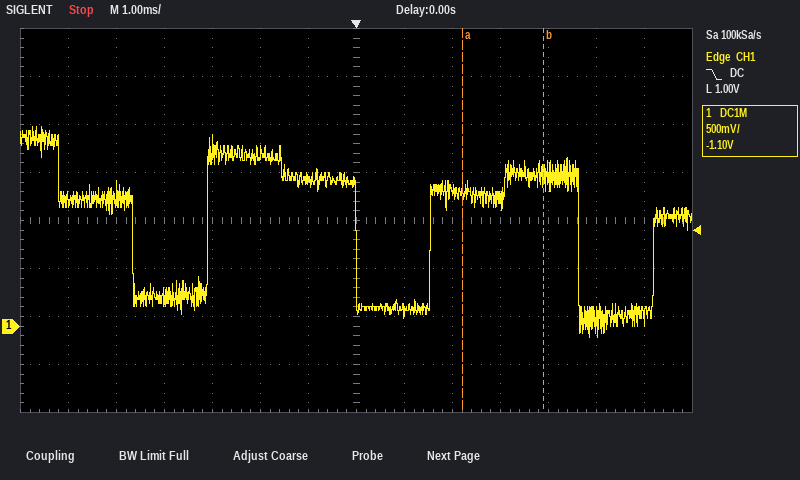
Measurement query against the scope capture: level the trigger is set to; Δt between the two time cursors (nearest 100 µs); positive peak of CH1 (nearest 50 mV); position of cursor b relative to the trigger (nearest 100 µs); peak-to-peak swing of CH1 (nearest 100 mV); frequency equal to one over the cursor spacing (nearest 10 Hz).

1.00 V
1.7 ms
2.10 V
+3.9 ms
2.20 V
590 Hz
